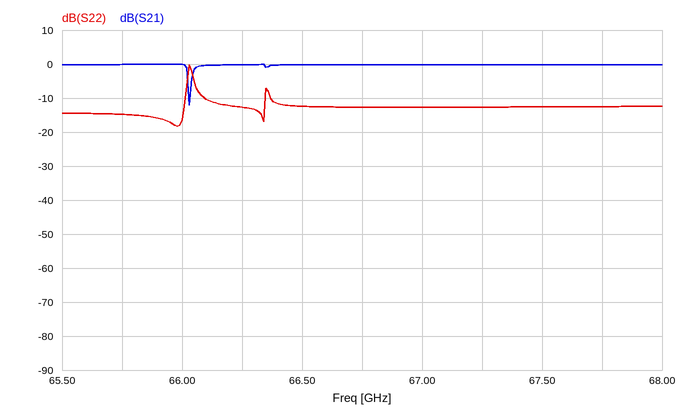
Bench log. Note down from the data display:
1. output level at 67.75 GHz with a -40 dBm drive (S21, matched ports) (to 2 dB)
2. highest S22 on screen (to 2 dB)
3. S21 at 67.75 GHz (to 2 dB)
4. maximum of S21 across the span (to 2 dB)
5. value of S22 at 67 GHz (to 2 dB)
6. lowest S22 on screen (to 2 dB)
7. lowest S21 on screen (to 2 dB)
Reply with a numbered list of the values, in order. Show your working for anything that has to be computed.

1. -40 dBm + (0 dB) = -40 dBm
2. 0 dB
3. 0 dB
4. 0 dB
5. -12 dB
6. -18 dB
7. -12 dB
